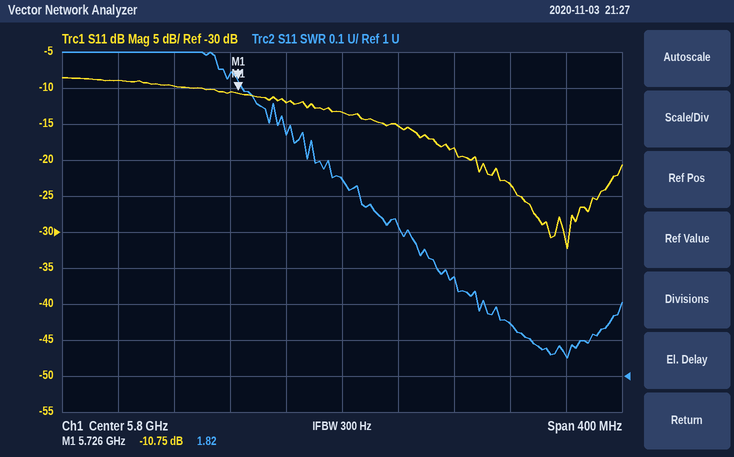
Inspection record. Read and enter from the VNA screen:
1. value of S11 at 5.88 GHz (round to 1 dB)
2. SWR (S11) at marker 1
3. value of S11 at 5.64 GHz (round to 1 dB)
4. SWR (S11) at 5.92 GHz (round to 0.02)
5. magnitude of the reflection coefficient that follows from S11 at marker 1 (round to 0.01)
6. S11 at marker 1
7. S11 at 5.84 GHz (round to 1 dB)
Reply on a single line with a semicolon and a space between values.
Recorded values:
-18 dB; 1.82; -9 dB; 1.14; 0.29; -10.75 dB; -15 dB
